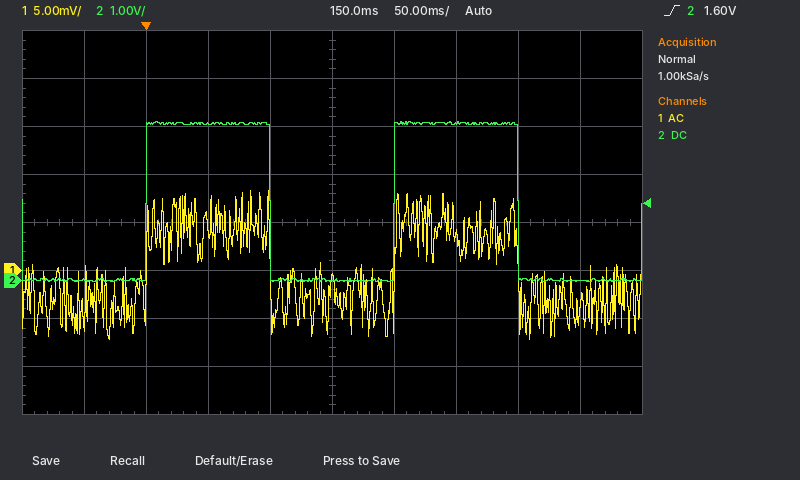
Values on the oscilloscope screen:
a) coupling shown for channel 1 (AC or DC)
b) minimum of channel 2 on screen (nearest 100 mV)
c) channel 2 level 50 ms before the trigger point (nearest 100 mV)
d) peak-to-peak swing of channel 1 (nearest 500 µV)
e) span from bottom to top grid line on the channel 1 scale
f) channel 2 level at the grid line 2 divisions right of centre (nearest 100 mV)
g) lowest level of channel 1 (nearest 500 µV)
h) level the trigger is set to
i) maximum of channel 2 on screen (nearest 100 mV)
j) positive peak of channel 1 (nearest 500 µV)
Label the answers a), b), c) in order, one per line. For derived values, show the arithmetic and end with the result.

a) AC
b) 0.0 V
c) 0.0 V
d) 8.5 mV − (-7.0 mV) = 15.5 mV
e) 40 mV
f) 3.3 V
g) -7.0 mV
h) 1.60 V
i) 3.3 V
j) 8.5 mV
